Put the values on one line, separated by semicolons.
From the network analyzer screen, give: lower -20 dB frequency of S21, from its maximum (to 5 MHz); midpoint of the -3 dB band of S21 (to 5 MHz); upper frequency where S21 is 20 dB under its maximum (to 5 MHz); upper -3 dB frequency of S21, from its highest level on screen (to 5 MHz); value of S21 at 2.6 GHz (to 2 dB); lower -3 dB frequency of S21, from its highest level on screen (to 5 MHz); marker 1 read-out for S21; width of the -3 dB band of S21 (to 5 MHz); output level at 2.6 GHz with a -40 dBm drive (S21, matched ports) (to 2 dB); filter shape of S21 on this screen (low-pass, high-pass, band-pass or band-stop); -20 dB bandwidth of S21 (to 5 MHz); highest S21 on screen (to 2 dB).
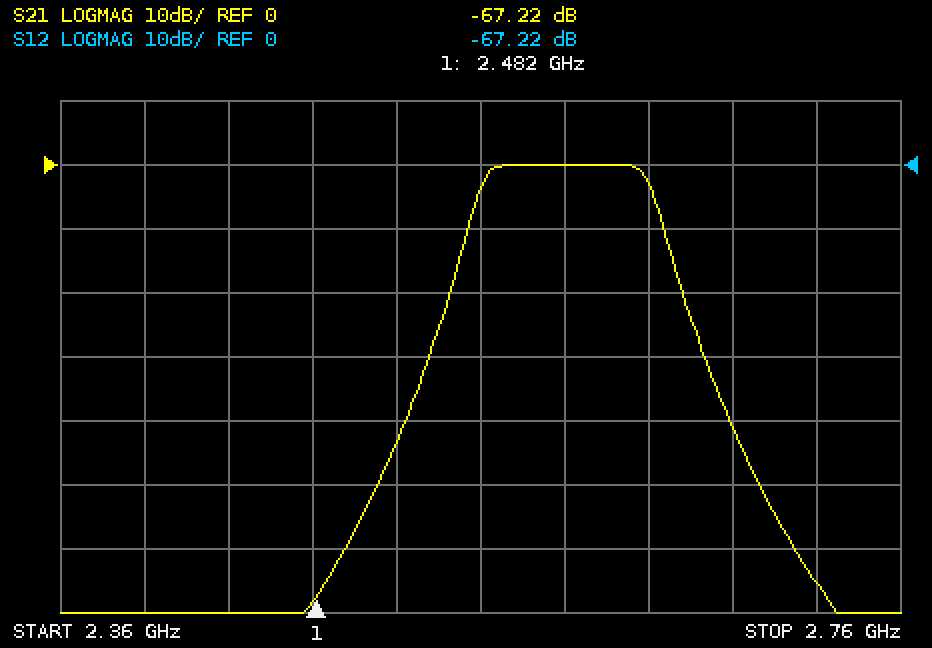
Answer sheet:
2.545 GHz; 2.600 GHz; 2.655 GHz; 2.640 GHz; 0 dB; 2.560 GHz; -67.22 dB; 80 MHz; -40 dBm; band-pass; 110 MHz; 0 dB
